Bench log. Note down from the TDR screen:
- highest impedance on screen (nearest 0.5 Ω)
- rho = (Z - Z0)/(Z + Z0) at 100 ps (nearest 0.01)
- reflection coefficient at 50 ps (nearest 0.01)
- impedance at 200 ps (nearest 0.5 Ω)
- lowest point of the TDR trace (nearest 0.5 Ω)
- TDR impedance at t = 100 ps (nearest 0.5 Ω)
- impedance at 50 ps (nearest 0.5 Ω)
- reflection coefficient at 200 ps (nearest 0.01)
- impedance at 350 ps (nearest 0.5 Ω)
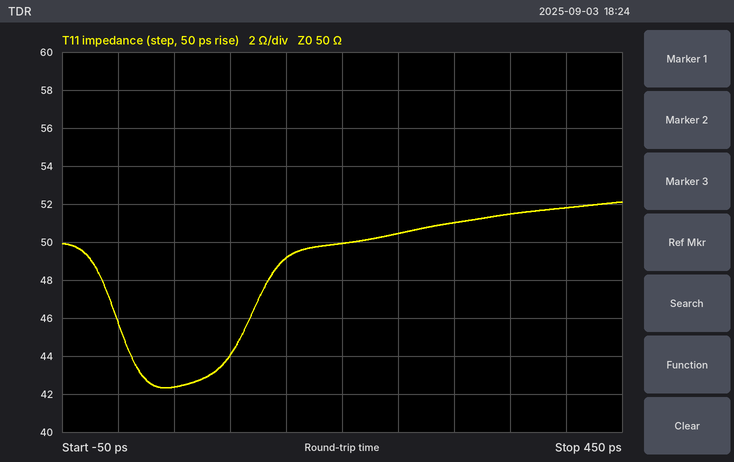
52.0 Ω
-0.06
-0.08
50.0 Ω
42.5 Ω
44.0 Ω
42.5 Ω
0.00
51.5 Ω
